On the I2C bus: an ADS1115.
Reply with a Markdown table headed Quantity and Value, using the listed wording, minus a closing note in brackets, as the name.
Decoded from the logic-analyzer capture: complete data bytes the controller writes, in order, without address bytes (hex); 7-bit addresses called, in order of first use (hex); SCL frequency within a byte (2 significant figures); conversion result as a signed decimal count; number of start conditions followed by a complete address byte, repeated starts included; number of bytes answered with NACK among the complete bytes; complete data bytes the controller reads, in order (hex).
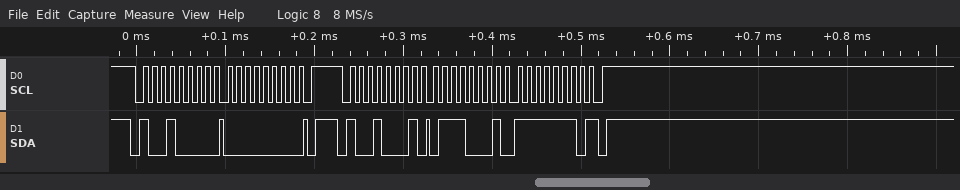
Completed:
| Quantity | Value |
|---|---|
| complete data bytes the controller writes, in order, without address bytes | 00 |
| 7-bit addresses called, in order of first use | 0x48 |
| SCL frequency within a byte | 100 kHz |
| conversion result as a signed decimal count | 29182 |
| number of start conditions followed by a complete address byte, repeated starts included | 2 |
| number of bytes answered with NACK among the complete bytes | 1 |
| complete data bytes the controller reads, in order | 71 FE |
